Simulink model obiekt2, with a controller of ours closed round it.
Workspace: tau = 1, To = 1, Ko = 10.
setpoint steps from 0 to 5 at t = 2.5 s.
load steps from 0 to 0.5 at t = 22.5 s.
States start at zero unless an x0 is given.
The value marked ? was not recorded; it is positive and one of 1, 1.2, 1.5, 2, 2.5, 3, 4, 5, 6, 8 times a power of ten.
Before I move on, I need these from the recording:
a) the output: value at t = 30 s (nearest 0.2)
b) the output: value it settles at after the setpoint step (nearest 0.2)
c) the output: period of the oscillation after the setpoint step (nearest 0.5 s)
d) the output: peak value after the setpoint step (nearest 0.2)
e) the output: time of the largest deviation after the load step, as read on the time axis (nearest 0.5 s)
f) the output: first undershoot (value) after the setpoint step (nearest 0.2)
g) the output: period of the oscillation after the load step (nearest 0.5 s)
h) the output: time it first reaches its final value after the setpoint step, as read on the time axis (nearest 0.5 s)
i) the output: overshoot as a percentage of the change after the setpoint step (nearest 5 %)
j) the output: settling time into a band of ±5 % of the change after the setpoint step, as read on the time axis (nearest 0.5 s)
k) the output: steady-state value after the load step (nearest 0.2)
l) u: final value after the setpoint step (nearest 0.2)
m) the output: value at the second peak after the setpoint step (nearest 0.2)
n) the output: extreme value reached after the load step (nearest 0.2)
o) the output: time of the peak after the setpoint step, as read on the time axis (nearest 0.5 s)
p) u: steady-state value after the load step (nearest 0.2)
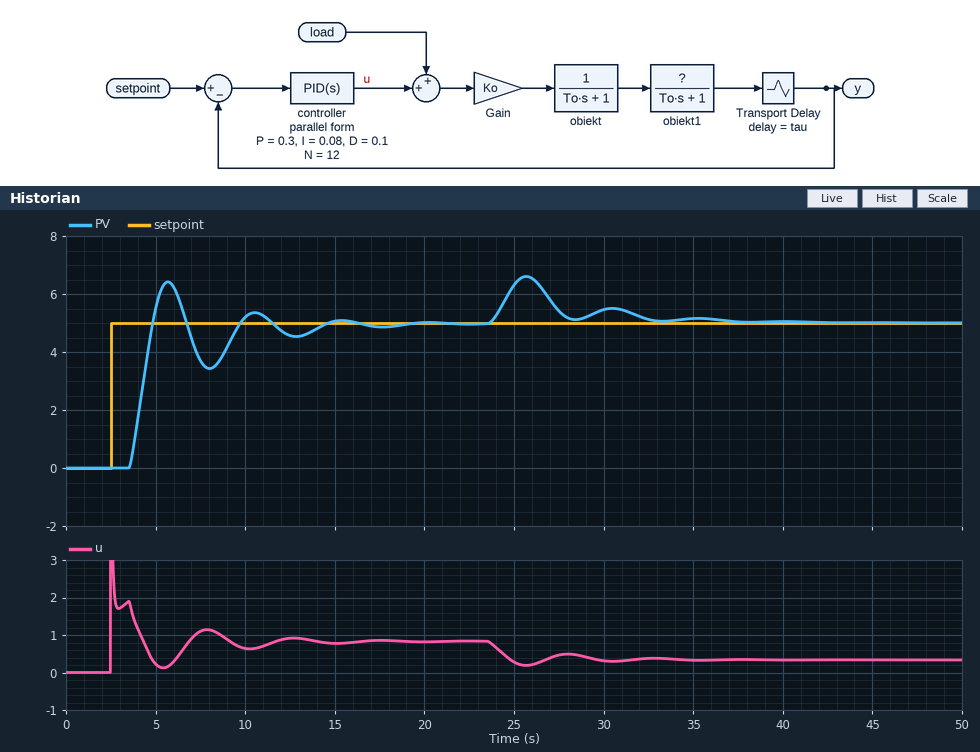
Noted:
5.4
5.0
5.0 s
6.4
25.5 s
3.4
5.0 s
5.0 s
30 %
14.0 s
5.0
0.8
5.4
6.6
5.5 s
0.4
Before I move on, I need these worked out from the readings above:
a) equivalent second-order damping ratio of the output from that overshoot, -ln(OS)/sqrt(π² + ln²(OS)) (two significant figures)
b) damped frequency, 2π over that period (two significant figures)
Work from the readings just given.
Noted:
0.36
1.3 rad/s
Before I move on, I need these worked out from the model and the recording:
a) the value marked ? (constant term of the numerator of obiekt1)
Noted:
0.6
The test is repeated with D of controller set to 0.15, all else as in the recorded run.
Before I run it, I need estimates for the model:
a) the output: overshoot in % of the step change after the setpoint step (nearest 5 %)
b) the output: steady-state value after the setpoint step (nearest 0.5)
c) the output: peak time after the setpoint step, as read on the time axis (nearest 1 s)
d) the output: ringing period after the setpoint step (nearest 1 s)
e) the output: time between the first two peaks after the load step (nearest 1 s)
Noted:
25 %
5.0
5 s
4 s
4 s
